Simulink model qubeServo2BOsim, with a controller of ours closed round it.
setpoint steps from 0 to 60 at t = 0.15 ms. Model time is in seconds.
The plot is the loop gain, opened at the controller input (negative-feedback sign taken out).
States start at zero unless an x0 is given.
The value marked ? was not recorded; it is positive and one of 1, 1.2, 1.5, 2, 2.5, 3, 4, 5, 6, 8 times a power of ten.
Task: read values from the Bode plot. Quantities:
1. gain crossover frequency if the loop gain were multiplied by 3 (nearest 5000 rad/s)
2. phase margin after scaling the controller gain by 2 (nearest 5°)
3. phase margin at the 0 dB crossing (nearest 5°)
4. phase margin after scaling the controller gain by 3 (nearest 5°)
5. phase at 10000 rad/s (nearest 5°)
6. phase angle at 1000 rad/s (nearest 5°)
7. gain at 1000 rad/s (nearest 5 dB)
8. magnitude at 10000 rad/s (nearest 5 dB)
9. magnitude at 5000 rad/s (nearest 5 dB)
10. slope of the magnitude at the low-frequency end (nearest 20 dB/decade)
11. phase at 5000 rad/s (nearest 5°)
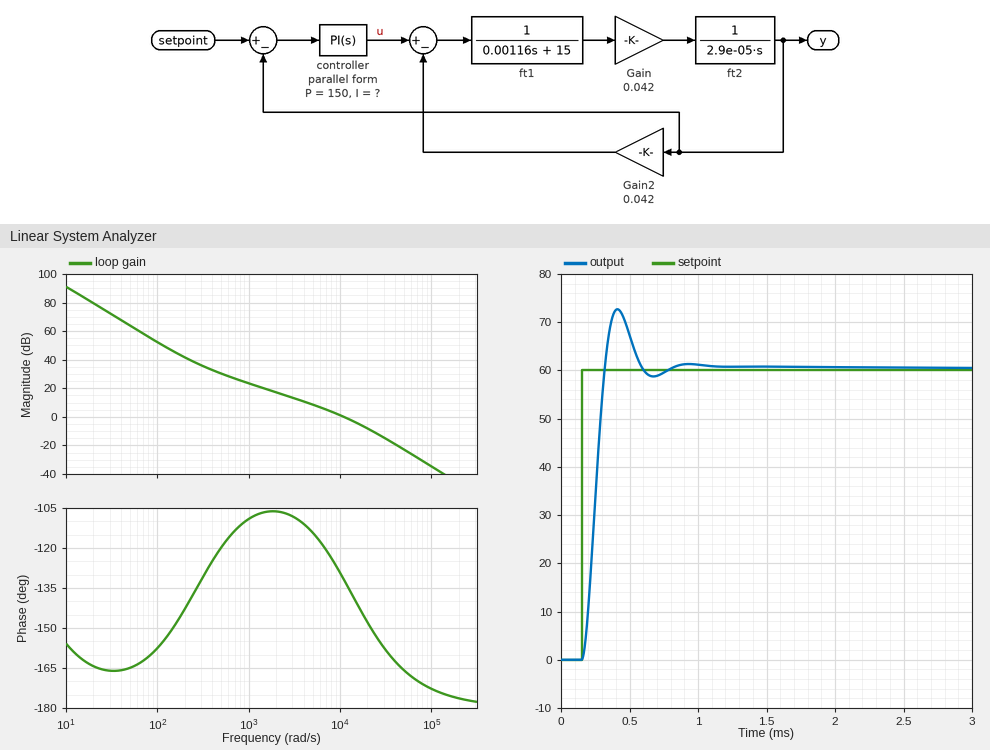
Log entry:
20000 rad/s
35°
50°
30°
-130°
-110°
25 dB
0 dB
10 dB
-40 dB/decade
-115°
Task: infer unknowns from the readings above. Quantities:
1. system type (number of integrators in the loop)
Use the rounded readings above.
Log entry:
2
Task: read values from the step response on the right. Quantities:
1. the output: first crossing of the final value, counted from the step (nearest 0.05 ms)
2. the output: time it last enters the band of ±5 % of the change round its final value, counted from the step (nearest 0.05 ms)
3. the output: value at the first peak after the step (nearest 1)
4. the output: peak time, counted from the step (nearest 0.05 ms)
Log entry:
0.15 ms
0.40 ms
73
0.25 ms
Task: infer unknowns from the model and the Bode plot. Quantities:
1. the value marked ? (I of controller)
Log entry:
40000
